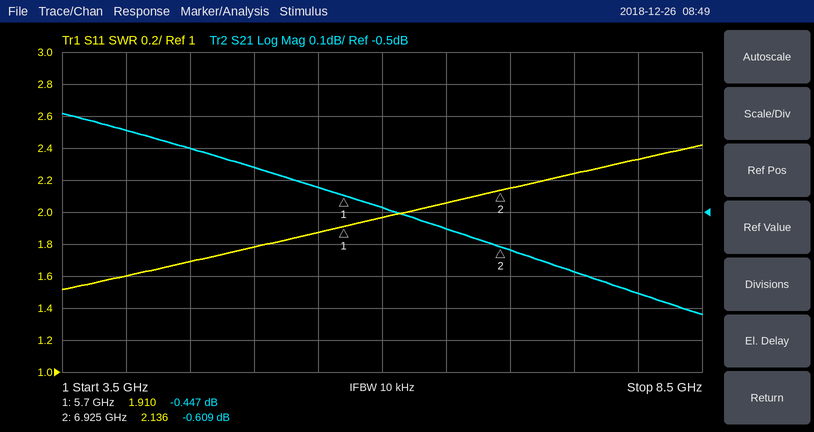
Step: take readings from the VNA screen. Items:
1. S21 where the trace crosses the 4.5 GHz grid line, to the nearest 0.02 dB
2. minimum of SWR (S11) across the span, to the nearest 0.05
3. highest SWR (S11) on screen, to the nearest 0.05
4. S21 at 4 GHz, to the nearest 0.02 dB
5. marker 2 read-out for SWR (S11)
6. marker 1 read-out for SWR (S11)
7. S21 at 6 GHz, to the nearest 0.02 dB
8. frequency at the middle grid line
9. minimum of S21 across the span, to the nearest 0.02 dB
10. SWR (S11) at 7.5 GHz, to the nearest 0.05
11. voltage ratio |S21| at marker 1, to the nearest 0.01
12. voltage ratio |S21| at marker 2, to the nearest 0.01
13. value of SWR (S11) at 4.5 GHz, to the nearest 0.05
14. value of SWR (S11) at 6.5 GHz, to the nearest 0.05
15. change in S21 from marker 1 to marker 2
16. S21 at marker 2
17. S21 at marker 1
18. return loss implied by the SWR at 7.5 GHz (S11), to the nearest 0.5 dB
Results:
-0.30 dB
1.50
2.40
-0.24 dB
2.136
1.910
-0.48 dB
6 GHz
-0.82 dB
2.25
0.95
0.93
1.70
2.05
-0.162 dB
-0.609 dB
-0.447 dB
8.5 dB
